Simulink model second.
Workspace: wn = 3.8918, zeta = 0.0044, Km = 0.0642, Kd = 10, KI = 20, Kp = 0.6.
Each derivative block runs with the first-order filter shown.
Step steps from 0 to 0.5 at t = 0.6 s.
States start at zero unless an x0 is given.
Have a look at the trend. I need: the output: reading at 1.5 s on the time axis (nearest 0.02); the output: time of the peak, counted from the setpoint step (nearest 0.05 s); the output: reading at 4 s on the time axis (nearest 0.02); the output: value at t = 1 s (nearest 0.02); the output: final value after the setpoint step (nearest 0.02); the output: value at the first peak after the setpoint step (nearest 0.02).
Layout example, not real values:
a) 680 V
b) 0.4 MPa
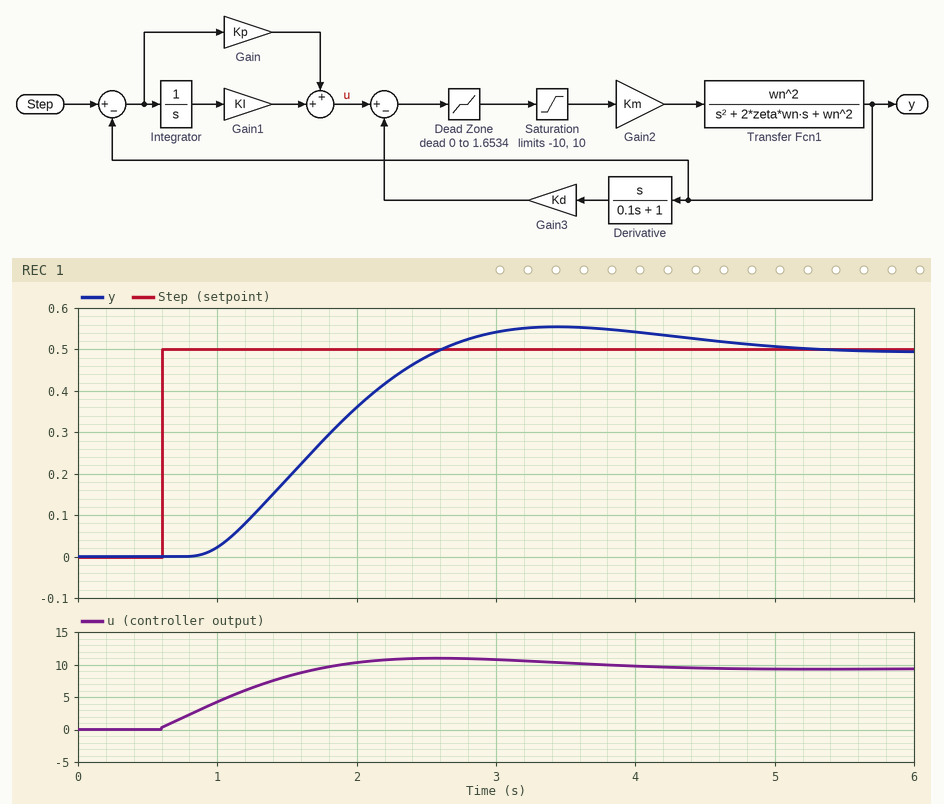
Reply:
a) 0.18
b) 2.85 s
c) 0.54
d) 0.02
e) 0.50
f) 0.56
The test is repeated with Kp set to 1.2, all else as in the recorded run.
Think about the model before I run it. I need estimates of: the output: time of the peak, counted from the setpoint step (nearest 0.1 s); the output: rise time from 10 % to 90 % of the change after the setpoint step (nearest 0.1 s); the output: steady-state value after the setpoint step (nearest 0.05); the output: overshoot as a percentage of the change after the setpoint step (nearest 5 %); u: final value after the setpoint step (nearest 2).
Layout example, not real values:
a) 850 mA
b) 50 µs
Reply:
a) 2.9 s
b) 1.3 s
c) 0.50
d) 10 %
e) 10
